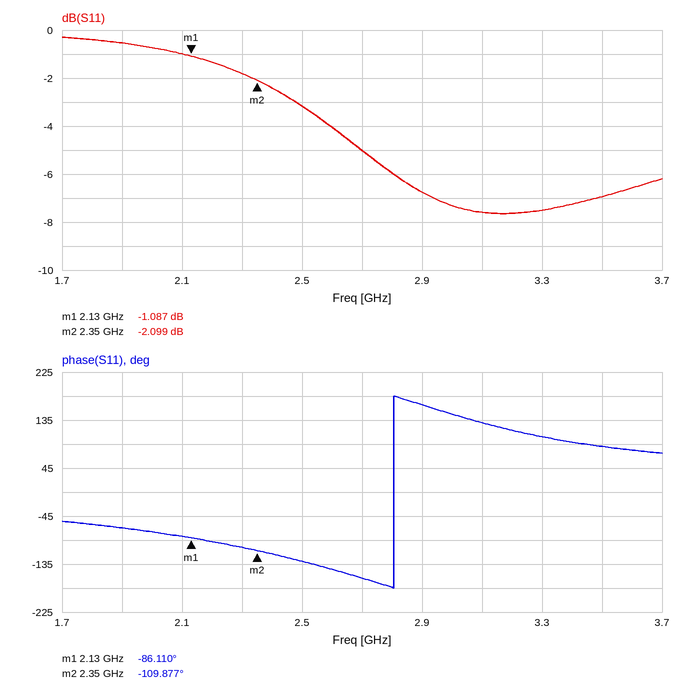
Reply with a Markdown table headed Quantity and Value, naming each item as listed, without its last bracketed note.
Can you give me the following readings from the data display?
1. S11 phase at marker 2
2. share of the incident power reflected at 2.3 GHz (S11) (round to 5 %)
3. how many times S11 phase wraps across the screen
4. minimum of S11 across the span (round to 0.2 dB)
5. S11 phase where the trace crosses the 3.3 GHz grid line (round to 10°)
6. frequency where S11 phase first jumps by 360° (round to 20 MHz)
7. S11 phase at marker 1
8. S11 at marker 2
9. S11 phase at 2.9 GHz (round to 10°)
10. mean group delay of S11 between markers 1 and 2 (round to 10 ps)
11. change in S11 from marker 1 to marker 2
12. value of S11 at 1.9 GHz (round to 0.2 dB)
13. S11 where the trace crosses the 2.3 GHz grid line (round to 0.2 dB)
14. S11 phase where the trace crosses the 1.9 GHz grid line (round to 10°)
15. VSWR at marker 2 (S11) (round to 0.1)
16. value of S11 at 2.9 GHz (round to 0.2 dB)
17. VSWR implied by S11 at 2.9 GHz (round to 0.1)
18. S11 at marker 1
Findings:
| Quantity | Value |
|---|---|
| S11 phase at marker 2 | -109.877° |
| share of the incident power reflected at 2.3 GHz (S11) | 65 % |
| how many times S11 phase wraps across the screen | 1 |
| minimum of S11 across the span | -7.6 dB |
| S11 phase where the trace crosses the 3.3 GHz grid line | 100° |
| frequency where S11 phase first jumps by 360° | 2.80 GHz |
| S11 phase at marker 1 | -86.110° |
| S11 at marker 2 | -2.099 dB |
| S11 phase at 2.9 GHz | 160° |
| mean group delay of S11 between markers 1 and 2 | 300 ps |
| change in S11 from marker 1 to marker 2 | -1.012 dB |
| value of S11 at 1.9 GHz | -0.6 dB |
| S11 where the trace crosses the 2.3 GHz grid line | -1.8 dB |
| S11 phase where the trace crosses the 1.9 GHz grid line | -70° |
| VSWR at marker 2 (S11) | 8.3 |
| value of S11 at 2.9 GHz | -6.8 dB |
| VSWR implied by S11 at 2.9 GHz | 2.7 |
| S11 at marker 1 | -1.087 dB |
